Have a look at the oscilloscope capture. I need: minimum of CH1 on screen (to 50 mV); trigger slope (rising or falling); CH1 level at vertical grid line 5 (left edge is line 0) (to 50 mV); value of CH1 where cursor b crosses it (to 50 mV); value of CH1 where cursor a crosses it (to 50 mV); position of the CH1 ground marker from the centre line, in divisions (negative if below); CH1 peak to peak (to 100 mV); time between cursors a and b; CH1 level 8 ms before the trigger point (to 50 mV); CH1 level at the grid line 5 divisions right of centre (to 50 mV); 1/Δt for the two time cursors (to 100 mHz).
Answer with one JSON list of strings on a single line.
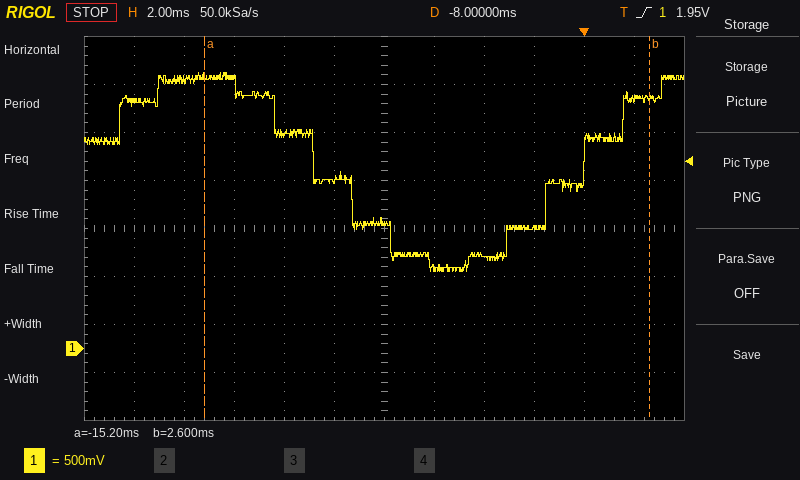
["800 mV", "rising", "1.75 V", "2.60 V", "2.85 V", "-2.5 div", "2.10 V", "17.8 ms", "1.30 V", "2.60 V", "56.2 Hz"]
